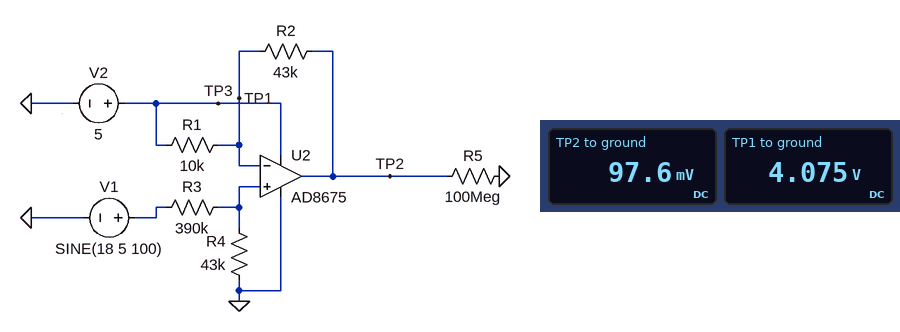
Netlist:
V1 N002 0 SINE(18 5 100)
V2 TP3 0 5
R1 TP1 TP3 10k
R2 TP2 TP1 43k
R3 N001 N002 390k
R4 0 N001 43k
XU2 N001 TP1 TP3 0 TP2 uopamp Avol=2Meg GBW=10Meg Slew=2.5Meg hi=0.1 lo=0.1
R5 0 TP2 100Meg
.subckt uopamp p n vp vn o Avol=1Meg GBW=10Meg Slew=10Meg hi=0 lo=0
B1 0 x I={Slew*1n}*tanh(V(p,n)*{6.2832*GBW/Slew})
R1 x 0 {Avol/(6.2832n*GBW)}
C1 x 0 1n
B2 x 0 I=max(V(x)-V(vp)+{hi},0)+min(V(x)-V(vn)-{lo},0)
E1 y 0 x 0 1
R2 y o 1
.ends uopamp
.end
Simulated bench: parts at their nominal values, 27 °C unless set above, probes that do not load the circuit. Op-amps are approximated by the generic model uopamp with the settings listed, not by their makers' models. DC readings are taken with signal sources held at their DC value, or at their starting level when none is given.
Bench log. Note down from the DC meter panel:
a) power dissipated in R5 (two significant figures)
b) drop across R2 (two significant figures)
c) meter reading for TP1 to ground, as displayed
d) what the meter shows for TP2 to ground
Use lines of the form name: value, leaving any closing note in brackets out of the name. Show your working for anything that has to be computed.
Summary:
power dissipated in R5: (97.6 mV)^2 / 100 MΩ = 95 pW
drop across R2: 4.075 V - 97.6 mV = 4.0 V
meter reading for TP1 to ground, as displayed: 4.075 V
what the meter shows for TP2 to ground: 97.6 mV
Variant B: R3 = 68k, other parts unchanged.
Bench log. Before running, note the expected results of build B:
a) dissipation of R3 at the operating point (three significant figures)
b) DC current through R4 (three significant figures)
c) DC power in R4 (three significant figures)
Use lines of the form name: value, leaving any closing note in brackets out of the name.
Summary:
dissipation of R3 at the operating point: 1.79 mW
DC current through R4: 162 µA
DC power in R4: 1.13 mW
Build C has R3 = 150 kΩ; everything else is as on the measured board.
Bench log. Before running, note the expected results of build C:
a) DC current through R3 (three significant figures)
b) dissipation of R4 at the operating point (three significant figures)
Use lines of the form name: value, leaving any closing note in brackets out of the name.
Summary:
DC current through R3: 93.3 µA
dissipation of R4 at the operating point: 374 µW
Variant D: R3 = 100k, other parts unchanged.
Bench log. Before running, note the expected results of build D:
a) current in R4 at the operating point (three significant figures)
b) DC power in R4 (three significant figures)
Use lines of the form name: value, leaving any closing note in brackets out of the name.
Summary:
current in R4 at the operating point: 126 µA
DC power in R4: 681 µW
